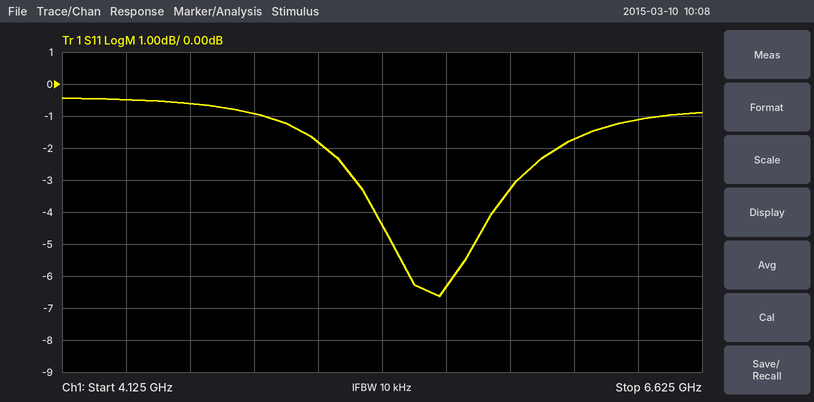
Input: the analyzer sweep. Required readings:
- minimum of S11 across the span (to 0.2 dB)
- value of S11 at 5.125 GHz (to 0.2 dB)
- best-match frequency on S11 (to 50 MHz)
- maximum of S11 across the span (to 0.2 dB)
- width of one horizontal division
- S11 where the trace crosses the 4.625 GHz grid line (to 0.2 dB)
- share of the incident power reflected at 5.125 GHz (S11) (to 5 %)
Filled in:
-6.6 dB
-1.8 dB
5.60 GHz
-0.4 dB
250 MHz
-0.6 dB
65 %
